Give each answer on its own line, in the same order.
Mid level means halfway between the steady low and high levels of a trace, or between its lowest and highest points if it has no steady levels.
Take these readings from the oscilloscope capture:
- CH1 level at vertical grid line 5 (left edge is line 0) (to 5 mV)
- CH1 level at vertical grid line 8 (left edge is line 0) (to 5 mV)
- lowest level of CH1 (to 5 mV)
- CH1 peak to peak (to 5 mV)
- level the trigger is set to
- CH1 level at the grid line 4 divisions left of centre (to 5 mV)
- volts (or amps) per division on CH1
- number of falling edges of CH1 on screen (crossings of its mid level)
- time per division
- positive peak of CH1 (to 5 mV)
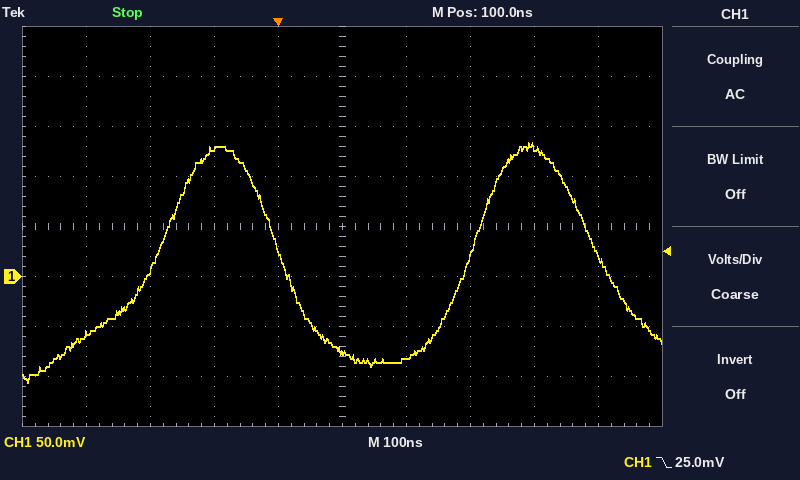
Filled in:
-75 mV
130 mV
-105 mV
240 mV
25.0 mV
-60 mV
50 mV
2
100 ns
135 mV
